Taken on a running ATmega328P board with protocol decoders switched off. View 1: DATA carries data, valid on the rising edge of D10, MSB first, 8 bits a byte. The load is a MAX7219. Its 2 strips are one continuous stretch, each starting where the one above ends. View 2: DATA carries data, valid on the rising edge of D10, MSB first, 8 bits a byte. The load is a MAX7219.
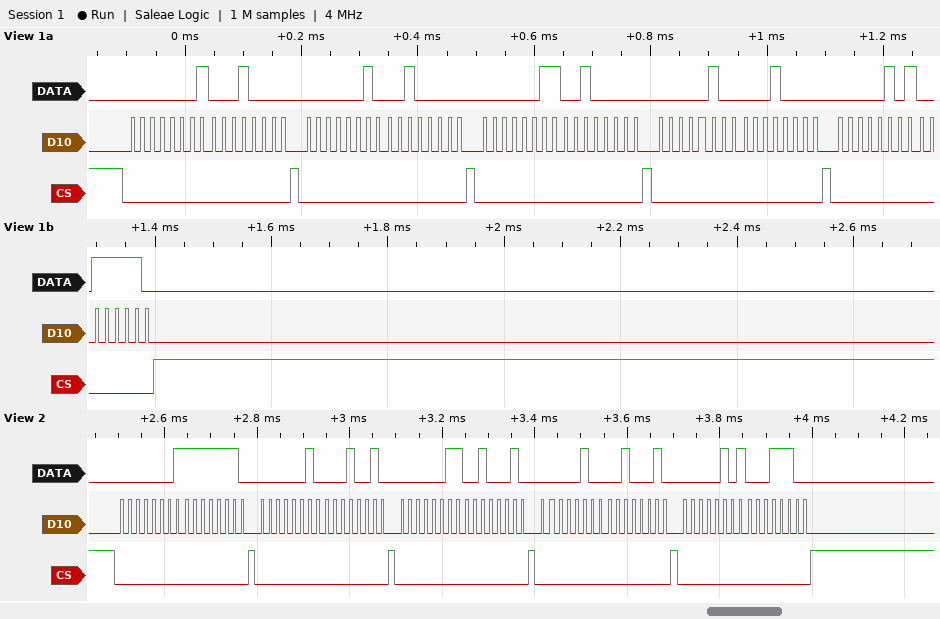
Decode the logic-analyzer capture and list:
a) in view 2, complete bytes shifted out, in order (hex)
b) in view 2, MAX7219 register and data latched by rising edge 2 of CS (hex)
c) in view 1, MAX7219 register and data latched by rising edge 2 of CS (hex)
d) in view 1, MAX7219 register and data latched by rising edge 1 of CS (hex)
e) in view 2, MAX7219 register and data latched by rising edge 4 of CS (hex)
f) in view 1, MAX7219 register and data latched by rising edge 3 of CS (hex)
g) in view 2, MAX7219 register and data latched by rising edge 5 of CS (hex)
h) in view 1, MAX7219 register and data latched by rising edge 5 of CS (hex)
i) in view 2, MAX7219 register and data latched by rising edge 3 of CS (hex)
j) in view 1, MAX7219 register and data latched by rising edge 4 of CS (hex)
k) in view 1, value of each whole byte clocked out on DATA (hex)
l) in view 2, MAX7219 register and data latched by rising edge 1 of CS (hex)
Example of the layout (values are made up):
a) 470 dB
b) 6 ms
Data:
a) 01 FE 02 12 03 22 04 22 05 1C
b) register 0x2, data 0x12
c) register 0x2, data 0x20
d) register 0x1, data 0x10
e) register 0x4, data 0x22
f) register 0x3, data 0x20
g) register 0x5, data 0x1C
h) register 0x5, data 0x3E
i) register 0x3, data 0x22
j) register 0x4, data 0x10
k) 01 10 02 20 03 20 04 10 05 3E
l) register 0x1, data 0xFE
